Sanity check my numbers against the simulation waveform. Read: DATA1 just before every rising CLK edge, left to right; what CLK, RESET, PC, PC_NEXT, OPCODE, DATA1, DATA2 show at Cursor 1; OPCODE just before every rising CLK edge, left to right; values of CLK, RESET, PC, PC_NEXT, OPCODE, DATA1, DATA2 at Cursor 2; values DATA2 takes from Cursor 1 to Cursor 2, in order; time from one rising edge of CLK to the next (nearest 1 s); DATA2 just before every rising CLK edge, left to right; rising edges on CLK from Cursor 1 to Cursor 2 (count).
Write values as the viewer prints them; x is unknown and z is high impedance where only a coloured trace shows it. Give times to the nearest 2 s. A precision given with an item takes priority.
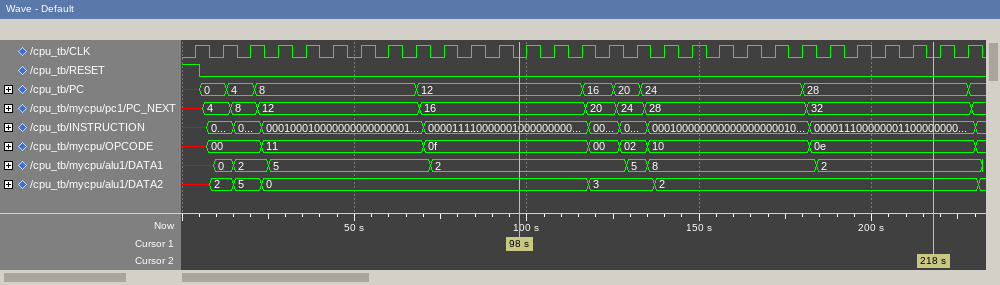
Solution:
x, 0, 2, 5, 5, 5, 5, 5, 5, 2, 2, 2, 2, 2, 2, 2, 5, 8, 8, 8, 8, 8, 8, 2, 2, 2, 2, 2, 2
CLK=0, RESET=0, PC=12, PC_NEXT=16, OPCODE=0f, DATA1=2, DATA2=0
x, 00, 00, 11, 11, 11, 11, 11, 11, 0f, 0f, 0f, 0f, 0f, 0f, 00, 02, 10, 10, 10, 10, 10, 10, 0e, 0e, 0e, 0e, 0e, 0e
CLK=0, RESET=0, PC=28, PC_NEXT=32, OPCODE=0e, DATA1=2, DATA2=2
0, 3, 2
8 s
x, 2, 5, 0, 0, 0, 0, 0, 0, 0, 0, 0, 0, 0, 0, 3, 3, 2, 2, 2, 2, 2, 2, 2, 2, 2, 2, 2, 2
15
